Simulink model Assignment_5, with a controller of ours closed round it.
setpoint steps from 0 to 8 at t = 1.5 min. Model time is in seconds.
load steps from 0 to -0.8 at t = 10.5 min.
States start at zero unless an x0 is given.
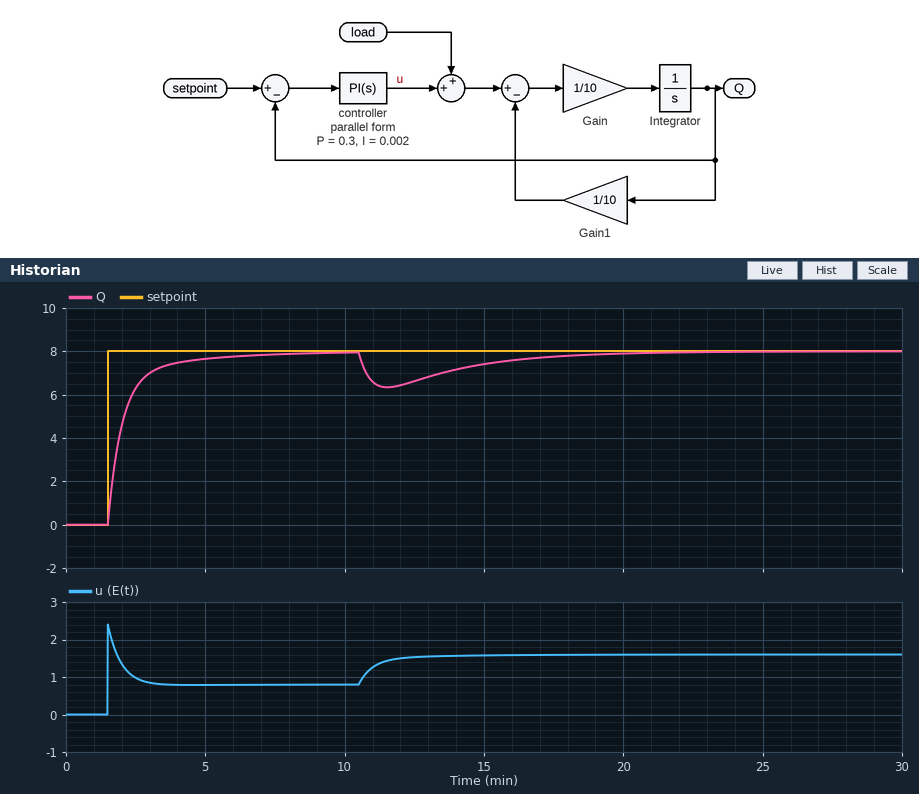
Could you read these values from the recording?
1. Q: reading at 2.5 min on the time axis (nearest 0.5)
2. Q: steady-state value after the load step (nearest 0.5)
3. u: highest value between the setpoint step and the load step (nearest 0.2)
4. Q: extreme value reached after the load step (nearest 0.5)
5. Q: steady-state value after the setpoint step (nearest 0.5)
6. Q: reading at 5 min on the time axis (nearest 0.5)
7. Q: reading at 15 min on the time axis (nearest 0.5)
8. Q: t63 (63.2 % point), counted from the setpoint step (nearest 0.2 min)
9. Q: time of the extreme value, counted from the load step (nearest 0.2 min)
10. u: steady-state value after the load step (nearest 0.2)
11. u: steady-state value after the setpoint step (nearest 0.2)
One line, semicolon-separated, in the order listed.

6.5; 8.0; 2.4; 6.5; 8.0; 7.5; 7.5; 0.6 min; 1.0 min; 1.6; 0.8
